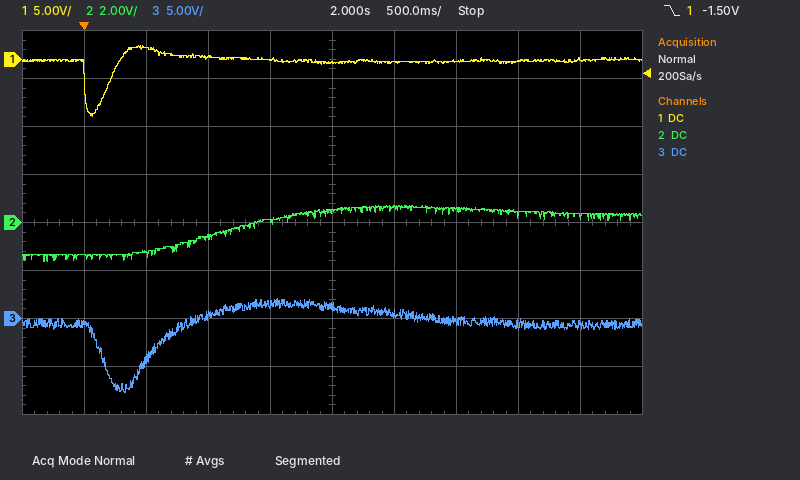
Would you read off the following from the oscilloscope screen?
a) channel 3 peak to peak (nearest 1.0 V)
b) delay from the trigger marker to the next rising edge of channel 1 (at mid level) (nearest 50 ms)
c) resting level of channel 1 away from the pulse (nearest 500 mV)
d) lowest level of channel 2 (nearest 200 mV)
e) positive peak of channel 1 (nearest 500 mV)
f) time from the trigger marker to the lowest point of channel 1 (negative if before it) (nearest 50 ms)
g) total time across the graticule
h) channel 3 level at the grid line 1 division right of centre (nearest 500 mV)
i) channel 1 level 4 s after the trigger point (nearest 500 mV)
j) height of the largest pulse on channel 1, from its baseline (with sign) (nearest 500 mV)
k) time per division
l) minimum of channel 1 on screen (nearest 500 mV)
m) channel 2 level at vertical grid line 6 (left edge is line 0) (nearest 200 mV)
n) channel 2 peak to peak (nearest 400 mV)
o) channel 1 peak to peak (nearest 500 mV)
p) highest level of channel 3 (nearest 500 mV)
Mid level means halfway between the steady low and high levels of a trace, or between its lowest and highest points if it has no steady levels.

10.0 V
200 ms
0.0 V
-1.6 V
1.5 V
+50 ms
5 s
500 mV
0.0 V
-6.0 V
500 ms
-6.0 V
600 mV
2.4 V
7.5 V
2.0 V
